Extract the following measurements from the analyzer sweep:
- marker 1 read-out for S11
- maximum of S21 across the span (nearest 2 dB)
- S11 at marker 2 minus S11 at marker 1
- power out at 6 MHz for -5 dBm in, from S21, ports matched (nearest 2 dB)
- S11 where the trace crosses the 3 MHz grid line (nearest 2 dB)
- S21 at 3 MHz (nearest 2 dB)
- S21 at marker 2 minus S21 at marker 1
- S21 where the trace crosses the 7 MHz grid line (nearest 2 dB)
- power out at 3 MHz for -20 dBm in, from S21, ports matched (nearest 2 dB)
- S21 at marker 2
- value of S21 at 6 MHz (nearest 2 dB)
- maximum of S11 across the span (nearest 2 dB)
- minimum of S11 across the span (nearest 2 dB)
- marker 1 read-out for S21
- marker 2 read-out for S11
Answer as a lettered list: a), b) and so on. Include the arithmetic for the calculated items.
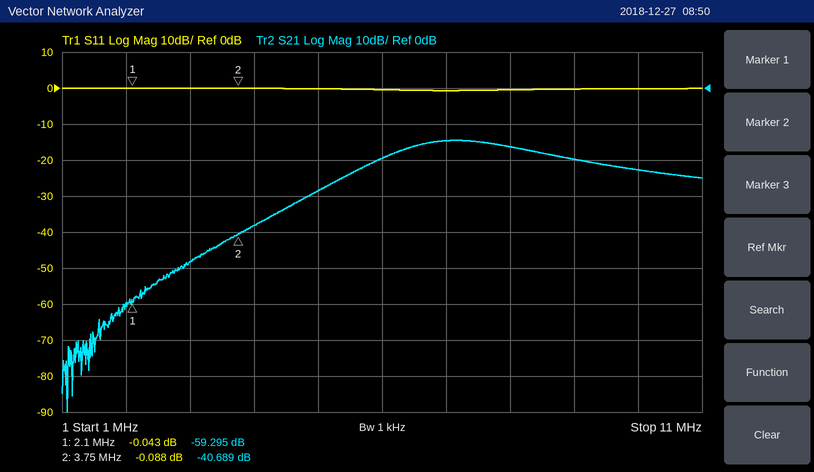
a) -0.043 dB
b) -14 dB
c) -0.088 − (-0.043) = -0.045 dB
d) -5 dBm + (-20 dB) = -24 dBm
e) 0 dB
f) -48 dB
g) -40.689 − (-59.295) = 18.606 dB
h) -14 dB
i) -20 dBm + (-48 dB) = -68 dBm
j) -40.689 dB
k) -20 dB
l) 0 dB
m) 0 dB
n) -59.295 dB
o) -0.088 dB
